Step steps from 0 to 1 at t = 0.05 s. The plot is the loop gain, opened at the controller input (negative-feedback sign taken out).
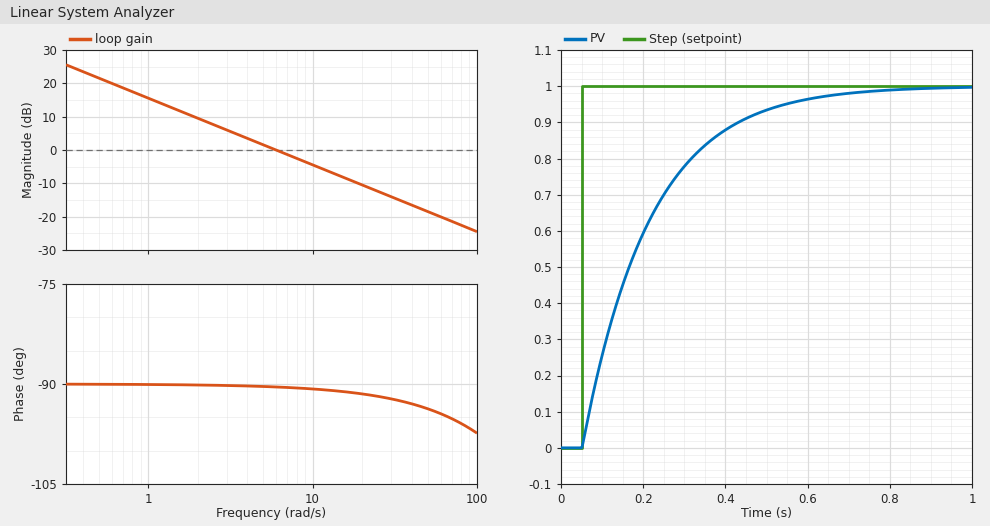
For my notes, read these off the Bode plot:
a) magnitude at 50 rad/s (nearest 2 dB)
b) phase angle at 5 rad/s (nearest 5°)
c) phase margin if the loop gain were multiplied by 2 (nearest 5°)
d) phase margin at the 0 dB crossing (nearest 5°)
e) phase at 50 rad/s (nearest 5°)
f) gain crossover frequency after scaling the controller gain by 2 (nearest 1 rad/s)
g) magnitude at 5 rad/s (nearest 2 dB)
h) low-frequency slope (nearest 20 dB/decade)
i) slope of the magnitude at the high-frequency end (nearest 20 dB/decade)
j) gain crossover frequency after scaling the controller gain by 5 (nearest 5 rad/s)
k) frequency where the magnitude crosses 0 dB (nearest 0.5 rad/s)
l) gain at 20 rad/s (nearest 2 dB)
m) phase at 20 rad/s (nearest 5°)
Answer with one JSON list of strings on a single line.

["-18 dB", "-90°", "90°", "90°", "-95°", "12 rad/s", "2 dB", "-20 dB/decade", "-20 dB/decade", "30 rad/s", "6.0 rad/s", "-10 dB", "-90°"]
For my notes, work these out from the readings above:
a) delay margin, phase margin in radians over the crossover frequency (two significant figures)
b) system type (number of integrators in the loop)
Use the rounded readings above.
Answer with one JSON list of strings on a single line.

["0.26 s", "1"]
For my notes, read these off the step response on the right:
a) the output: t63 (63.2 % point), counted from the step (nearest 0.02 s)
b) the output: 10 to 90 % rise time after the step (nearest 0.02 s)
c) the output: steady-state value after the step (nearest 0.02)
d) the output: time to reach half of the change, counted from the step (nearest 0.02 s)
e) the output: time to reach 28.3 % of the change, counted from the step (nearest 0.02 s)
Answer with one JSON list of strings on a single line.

["0.16 s", "0.36 s", "1.00", "0.12 s", "0.06 s"]
